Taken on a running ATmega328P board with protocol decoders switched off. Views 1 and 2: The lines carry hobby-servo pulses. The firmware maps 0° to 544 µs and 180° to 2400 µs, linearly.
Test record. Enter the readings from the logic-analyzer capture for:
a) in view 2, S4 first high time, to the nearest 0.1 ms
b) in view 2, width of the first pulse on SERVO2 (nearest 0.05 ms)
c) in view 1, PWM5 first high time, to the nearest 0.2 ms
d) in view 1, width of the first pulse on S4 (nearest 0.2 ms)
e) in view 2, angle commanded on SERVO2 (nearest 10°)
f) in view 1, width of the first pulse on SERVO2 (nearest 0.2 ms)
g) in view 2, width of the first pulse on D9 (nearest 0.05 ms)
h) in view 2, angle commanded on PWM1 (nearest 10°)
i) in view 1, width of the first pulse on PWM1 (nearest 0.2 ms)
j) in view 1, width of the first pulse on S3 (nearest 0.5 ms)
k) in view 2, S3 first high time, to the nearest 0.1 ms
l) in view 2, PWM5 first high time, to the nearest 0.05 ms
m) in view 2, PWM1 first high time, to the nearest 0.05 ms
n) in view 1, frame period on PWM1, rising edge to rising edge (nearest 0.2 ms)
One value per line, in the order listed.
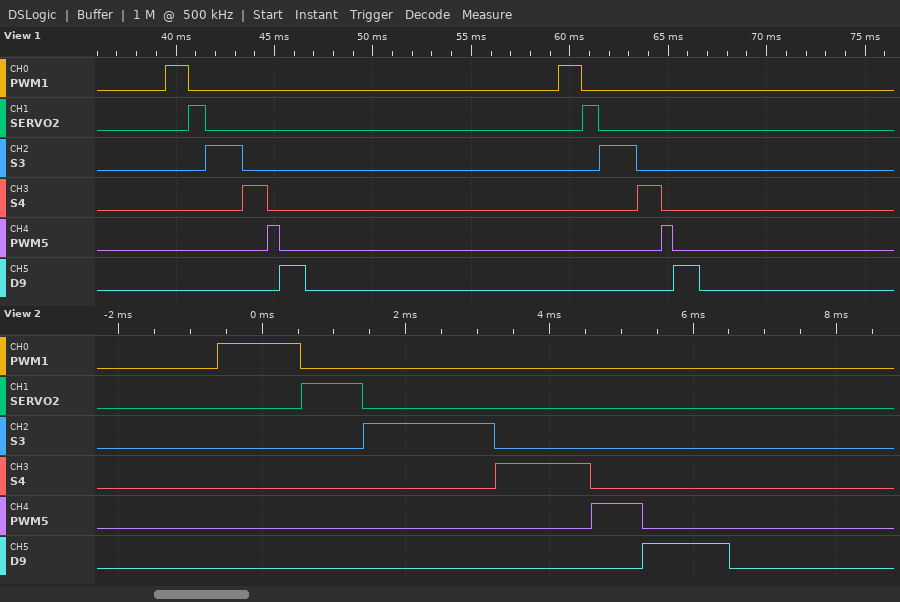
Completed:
1.3 ms
0.85 ms
0.6 ms
1.2 ms
30°
0.8 ms
1.20 ms
60°
1.2 ms
2.0 ms
1.8 ms
0.70 ms
1.15 ms
20.0 ms
